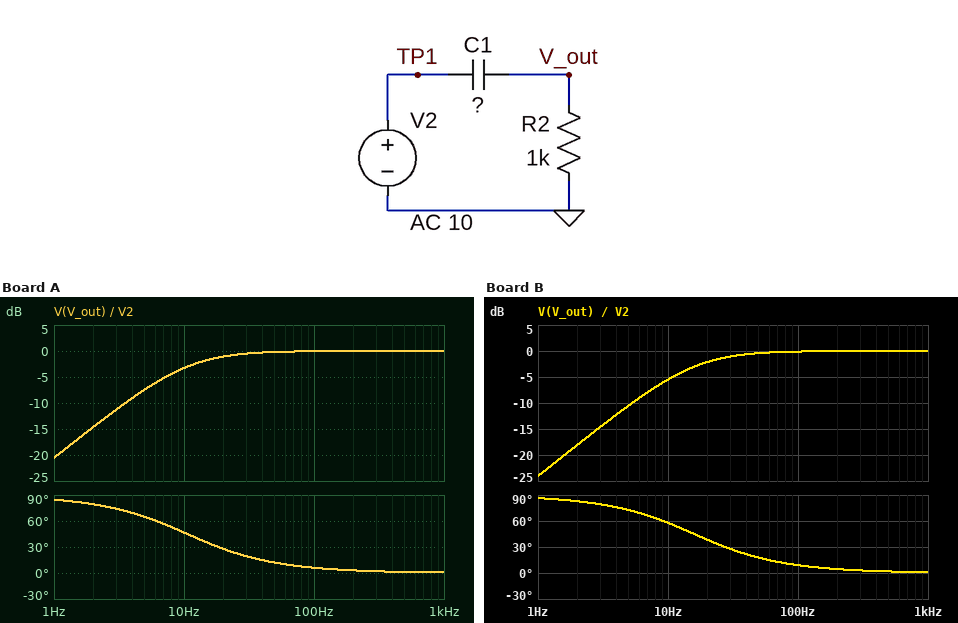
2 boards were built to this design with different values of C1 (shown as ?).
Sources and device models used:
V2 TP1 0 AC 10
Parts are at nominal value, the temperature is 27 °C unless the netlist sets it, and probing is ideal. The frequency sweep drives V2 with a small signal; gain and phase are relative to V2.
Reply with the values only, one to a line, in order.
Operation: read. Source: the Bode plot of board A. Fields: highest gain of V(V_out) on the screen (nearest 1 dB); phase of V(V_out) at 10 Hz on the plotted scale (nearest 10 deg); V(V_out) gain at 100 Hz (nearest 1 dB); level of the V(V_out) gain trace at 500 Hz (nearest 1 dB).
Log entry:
0 dB
50 deg
0 dB
0 dB
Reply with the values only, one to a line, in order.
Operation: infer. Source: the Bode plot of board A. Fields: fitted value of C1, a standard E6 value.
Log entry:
15 µF
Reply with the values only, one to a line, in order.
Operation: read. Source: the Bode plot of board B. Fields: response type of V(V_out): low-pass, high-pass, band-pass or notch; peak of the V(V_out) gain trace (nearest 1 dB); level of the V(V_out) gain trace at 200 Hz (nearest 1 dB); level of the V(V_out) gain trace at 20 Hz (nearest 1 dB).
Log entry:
high-pass
0 dB
0 dB
-2 dB
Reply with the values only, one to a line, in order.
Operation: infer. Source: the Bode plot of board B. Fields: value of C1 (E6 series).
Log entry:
10 µF
